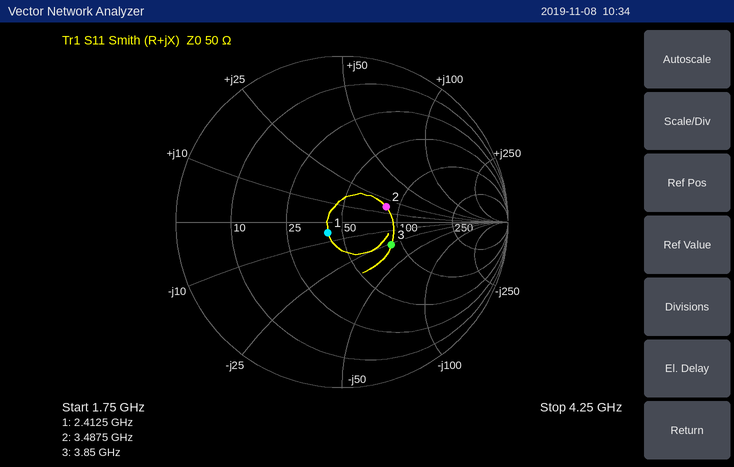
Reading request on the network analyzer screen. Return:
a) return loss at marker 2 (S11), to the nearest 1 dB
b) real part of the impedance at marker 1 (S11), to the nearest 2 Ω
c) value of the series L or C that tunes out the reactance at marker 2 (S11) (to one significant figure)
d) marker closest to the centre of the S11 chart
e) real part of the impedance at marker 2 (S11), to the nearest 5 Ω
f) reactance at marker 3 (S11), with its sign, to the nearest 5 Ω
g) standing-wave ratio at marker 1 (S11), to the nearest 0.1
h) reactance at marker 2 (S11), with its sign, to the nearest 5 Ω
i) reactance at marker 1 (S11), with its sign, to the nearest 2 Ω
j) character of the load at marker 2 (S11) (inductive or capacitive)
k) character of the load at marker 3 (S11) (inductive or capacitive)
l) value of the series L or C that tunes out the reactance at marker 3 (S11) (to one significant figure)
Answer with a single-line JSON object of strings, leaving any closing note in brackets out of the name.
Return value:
{"return loss at marker 2 (S11), to the nearest 1 dB": "11 dB", "real part of the impedance at marker 1 (S11), to the nearest 2 Ω": "42 Ω", "value of the series L or C that tunes out the reactance at marker 2 (S11)": "3 pF", "marker closest to the centre of the S11 chart": "marker 1", "real part of the impedance at marker 2 (S11), to the nearest 5 Ω": "85 Ω", "reactance at marker 3 (S11), with its sign, to the nearest 5 Ω": "-25 Ω", "standing-wave ratio at marker 1 (S11), to the nearest 0.1": "1.2", "reactance at marker 2 (S11), with its sign, to the nearest 5 Ω": "+15 Ω", "reactance at marker 1 (S11), with its sign, to the nearest 2 Ω": "-6 Ω", "character of the load at marker 2 (S11)": "inductive", "character of the load at marker 3 (S11)": "capacitive", "value of the series L or C that tunes out the reactance at marker 3 (S11)": "1 nH"}
